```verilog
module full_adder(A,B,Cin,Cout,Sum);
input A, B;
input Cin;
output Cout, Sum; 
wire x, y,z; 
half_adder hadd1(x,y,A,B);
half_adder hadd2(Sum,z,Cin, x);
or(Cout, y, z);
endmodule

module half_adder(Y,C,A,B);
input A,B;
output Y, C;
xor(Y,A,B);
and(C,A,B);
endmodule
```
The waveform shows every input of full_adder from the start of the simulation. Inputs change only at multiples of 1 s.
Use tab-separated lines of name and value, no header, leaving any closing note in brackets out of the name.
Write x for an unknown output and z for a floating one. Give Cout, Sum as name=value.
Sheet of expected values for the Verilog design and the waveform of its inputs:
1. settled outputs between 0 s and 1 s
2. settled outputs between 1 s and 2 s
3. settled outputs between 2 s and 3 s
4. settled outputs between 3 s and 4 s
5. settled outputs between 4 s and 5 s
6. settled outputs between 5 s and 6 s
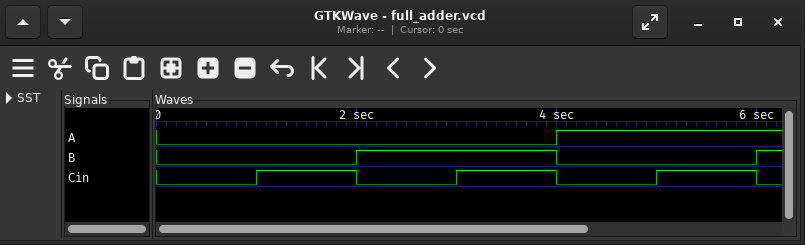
settled outputs between 0 s and 1 s	Cout=0, Sum=0
settled outputs between 1 s and 2 s	Cout=0, Sum=1
settled outputs between 2 s and 3 s	Cout=0, Sum=1
settled outputs between 3 s and 4 s	Cout=1, Sum=0
settled outputs between 4 s and 5 s	Cout=0, Sum=1
settled outputs between 5 s and 6 s	Cout=1, Sum=0
